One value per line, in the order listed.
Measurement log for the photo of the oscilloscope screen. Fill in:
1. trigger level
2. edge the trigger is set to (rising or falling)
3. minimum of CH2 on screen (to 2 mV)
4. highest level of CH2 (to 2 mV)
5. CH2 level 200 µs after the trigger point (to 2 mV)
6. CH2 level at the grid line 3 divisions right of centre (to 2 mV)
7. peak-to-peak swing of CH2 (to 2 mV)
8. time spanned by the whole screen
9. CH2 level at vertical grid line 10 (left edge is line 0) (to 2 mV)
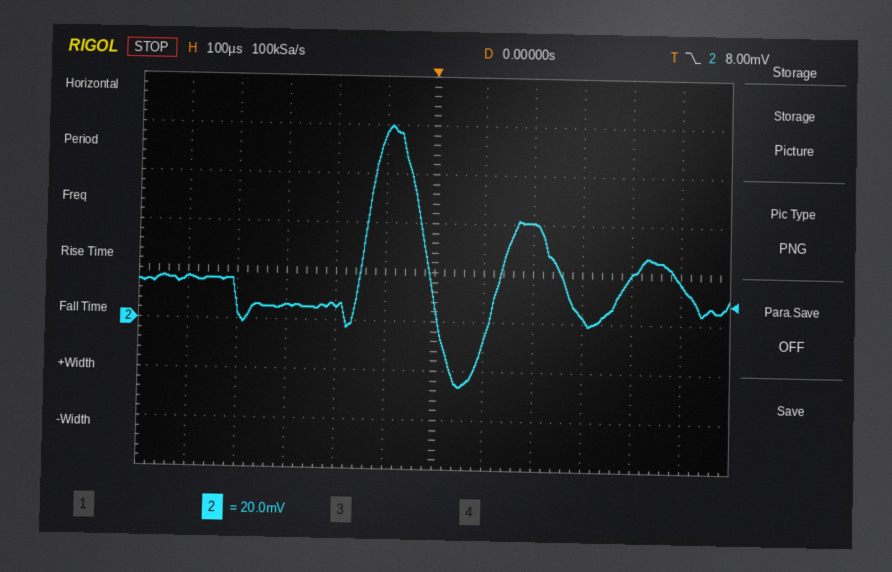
8.00 mV
falling
-26 mV
80 mV
40 mV
2 mV
106 mV
1.2 ms
20 mV
